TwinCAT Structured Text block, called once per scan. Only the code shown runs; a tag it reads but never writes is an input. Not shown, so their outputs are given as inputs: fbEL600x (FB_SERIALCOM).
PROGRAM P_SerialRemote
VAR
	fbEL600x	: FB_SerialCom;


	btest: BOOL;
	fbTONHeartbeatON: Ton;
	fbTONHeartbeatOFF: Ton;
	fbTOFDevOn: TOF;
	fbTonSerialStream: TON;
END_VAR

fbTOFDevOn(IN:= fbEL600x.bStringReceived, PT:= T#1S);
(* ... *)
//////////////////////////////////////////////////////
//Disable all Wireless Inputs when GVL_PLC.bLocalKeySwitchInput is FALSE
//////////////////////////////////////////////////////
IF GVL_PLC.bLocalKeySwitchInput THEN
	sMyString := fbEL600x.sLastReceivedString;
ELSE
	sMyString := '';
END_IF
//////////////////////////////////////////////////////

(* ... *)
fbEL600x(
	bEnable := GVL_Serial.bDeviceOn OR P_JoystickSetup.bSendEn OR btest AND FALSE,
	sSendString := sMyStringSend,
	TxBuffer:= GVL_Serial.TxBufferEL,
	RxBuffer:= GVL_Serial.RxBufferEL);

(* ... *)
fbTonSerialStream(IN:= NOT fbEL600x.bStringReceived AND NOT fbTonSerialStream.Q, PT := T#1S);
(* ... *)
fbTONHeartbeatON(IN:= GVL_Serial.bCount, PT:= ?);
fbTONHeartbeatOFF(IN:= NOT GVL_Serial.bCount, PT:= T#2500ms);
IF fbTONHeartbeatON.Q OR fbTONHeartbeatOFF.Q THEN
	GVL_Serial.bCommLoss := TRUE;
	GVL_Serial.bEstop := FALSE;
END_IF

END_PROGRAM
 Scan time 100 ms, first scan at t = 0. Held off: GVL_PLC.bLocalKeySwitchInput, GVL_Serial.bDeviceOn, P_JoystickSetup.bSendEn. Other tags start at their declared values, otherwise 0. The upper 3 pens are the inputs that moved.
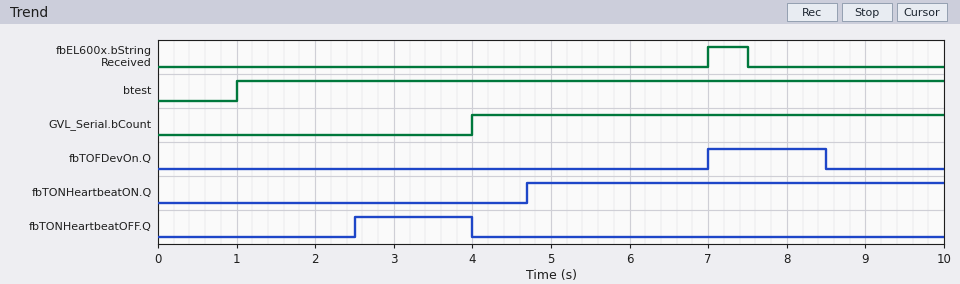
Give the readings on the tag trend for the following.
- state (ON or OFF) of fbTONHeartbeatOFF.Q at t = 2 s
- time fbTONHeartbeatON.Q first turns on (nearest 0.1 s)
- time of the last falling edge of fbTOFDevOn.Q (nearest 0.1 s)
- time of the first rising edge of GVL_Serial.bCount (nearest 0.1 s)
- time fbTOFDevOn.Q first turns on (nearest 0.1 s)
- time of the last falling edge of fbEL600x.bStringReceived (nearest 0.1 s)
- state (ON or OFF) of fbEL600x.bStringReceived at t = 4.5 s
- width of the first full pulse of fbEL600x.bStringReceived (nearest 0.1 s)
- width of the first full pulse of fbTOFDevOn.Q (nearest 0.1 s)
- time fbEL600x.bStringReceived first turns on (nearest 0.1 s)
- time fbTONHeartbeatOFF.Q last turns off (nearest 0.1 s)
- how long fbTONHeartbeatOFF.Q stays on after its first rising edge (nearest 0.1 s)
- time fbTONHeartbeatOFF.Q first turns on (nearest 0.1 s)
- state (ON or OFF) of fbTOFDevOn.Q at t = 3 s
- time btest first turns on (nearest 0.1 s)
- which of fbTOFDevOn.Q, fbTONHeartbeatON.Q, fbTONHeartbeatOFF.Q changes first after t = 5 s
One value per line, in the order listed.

OFF
4.7 s
8.5 s
4.0 s
7.0 s
7.5 s
OFF
0.5 s
1.5 s
7.0 s
4.0 s
1.5 s
2.5 s
OFF
1.0 s
fbTOFDevOn.Q
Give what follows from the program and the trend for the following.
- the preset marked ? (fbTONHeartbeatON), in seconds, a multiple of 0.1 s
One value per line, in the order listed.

0.7 s
